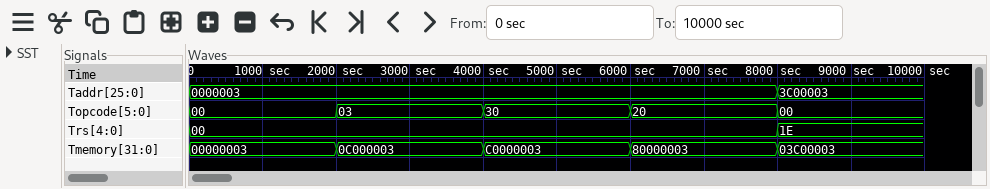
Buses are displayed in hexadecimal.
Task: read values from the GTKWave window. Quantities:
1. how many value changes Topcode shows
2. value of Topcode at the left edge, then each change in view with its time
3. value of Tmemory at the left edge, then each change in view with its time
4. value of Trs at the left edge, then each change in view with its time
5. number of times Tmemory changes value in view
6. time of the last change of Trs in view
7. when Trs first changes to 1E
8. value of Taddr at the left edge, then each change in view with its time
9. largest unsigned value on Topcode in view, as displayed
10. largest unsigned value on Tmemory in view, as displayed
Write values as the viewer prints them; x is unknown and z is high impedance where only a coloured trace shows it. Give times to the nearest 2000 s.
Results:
4
00, 03 at 2000 s, 30 at 4000 s, 20 at 6000 s, 00 at 8000 s
00000003, 0C000003 at 2000 s, C0000003 at 4000 s, 80000003 at 6000 s, 03C00003 at 8000 s
00, 1E at 8000 s
4
8000 s
8000 s
0000003, 3C00003 at 8000 s
30
C0000003
